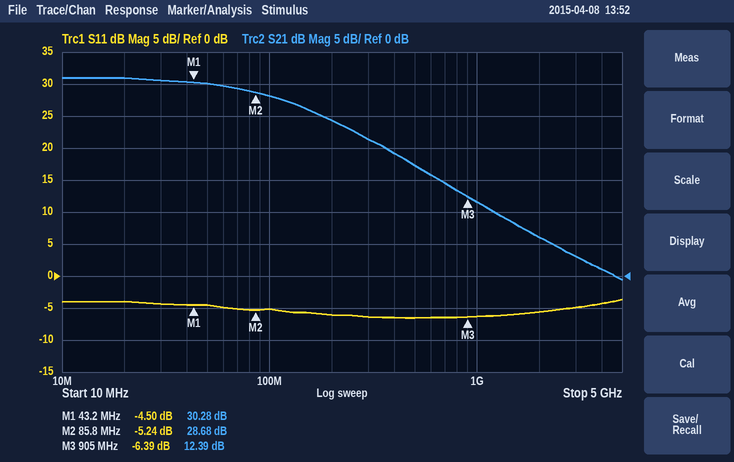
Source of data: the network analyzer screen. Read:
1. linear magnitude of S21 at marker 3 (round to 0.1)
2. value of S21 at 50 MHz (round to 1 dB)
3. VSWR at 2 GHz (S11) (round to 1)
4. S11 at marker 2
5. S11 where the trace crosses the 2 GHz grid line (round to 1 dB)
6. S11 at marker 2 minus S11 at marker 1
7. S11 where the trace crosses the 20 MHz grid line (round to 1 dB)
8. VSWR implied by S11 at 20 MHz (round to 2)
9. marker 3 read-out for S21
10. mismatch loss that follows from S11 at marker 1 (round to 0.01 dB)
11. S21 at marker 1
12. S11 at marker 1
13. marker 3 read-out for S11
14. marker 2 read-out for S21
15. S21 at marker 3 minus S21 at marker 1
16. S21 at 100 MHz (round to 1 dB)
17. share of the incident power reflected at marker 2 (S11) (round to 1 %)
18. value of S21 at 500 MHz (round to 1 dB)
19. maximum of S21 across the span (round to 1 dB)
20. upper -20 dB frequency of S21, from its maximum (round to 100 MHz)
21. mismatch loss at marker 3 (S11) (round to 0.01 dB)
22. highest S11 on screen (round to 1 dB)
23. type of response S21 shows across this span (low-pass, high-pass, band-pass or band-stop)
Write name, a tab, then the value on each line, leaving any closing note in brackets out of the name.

linear magnitude of S21 at marker 3	4.2
value of S21 at 50 MHz	30 dB
VSWR at 2 GHz (S11)	3
S11 at marker 2	-5.24 dB
S11 where the trace crosses the 2 GHz grid line	-6 dB
S11 at marker 2 minus S11 at marker 1	-0.74 dB
S11 where the trace crosses the 20 MHz grid line	-4 dB
VSWR implied by S11 at 20 MHz	4
marker 3 read-out for S21	12.39 dB
mismatch loss that follows from S11 at marker 1	1.90 dB
S21 at marker 1	30.28 dB
S11 at marker 1	-4.50 dB
marker 3 read-out for S11	-6.39 dB
marker 2 read-out for S21	28.68 dB
S21 at marker 3 minus S21 at marker 1	-17.89 dB
S21 at 100 MHz	28 dB
share of the incident power reflected at marker 2 (S11)	30 %
value of S21 at 500 MHz	17 dB
maximum of S21 across the span	31 dB
upper -20 dB frequency of S21, from its maximum	1.1 GHz
mismatch loss at marker 3 (S11)	1.13 dB
highest S11 on screen	-4 dB
type of response S21 shows across this span	low-pass
